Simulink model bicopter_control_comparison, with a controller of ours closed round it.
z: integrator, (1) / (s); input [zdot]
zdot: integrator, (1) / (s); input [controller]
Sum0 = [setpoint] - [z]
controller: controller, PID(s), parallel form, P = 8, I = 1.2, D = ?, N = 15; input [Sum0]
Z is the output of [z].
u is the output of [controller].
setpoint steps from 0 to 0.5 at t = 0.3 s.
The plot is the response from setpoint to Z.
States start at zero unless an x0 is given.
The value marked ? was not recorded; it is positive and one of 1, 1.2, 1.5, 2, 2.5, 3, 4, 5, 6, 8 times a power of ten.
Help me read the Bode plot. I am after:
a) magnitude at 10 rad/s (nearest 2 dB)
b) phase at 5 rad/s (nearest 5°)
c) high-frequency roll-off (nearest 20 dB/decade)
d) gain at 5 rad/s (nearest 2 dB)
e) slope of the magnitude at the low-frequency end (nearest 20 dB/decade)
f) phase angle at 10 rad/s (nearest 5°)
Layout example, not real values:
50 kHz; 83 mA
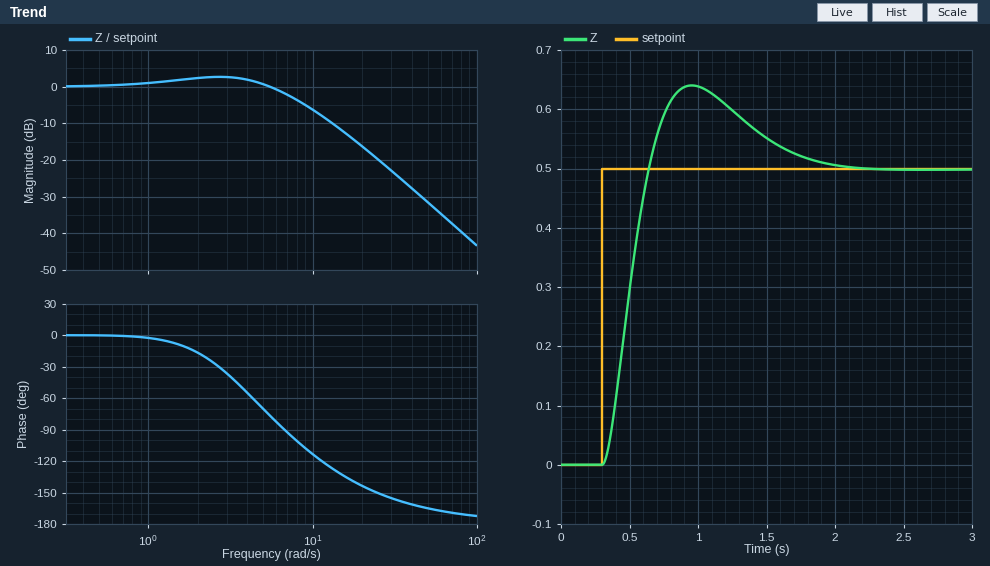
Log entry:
-6 dB; -70°; -40 dB/decade; 0 dB; 0 dB/decade; -115°
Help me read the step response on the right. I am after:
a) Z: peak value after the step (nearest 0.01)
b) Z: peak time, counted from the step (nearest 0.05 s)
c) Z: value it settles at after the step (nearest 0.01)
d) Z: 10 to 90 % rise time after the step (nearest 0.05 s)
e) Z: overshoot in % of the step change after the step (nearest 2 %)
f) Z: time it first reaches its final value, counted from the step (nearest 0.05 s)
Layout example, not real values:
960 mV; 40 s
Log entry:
0.64; 0.65 s; 0.50; 0.25 s; 28 %; 0.35 s
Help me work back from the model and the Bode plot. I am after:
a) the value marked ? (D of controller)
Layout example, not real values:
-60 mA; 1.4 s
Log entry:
4
